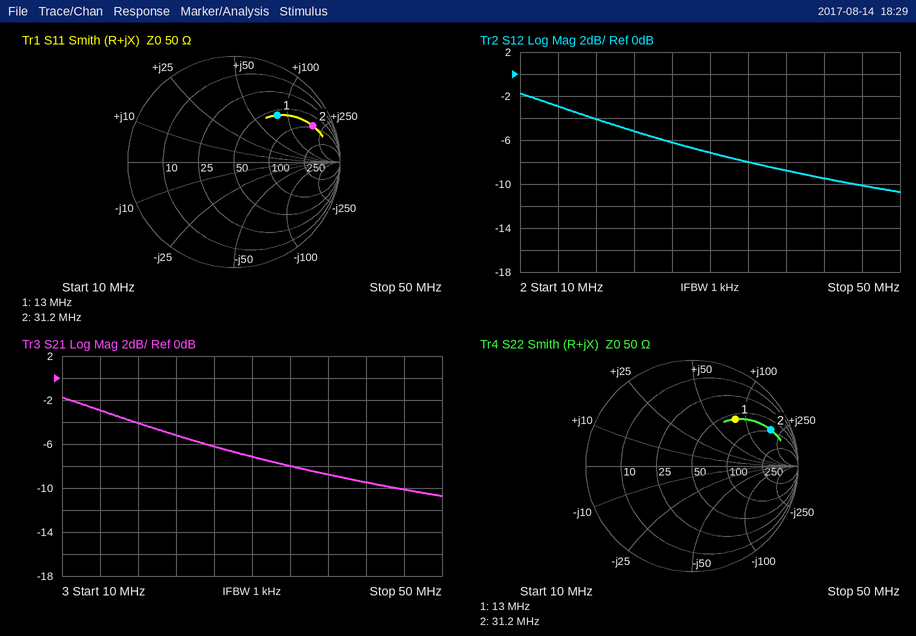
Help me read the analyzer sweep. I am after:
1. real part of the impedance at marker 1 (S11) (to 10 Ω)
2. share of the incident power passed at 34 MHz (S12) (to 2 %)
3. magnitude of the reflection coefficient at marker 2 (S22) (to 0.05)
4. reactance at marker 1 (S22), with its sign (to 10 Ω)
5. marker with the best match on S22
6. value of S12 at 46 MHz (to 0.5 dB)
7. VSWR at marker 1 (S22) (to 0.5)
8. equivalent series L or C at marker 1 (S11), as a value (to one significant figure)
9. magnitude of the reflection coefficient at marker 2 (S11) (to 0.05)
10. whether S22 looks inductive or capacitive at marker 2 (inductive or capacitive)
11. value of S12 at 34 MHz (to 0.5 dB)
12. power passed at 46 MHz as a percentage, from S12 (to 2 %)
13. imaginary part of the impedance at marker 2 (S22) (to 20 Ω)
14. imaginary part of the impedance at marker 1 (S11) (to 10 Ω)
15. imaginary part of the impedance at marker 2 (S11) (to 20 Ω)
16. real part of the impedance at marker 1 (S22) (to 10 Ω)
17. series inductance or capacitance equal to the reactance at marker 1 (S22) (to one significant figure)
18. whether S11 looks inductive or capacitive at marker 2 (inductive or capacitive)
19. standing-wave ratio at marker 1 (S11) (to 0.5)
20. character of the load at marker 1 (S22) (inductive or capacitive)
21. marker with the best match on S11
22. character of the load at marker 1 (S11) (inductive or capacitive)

60 Ω
16 %
0.80
+80 Ω
marker 1
-10.0 dB
4.0
1.0 µH
0.80
inductive
-8.0 dB
10 %
+180 Ω
+80 Ω
+180 Ω
60 Ω
1.0 µH
inductive
4.0
inductive
marker 1
inductive
